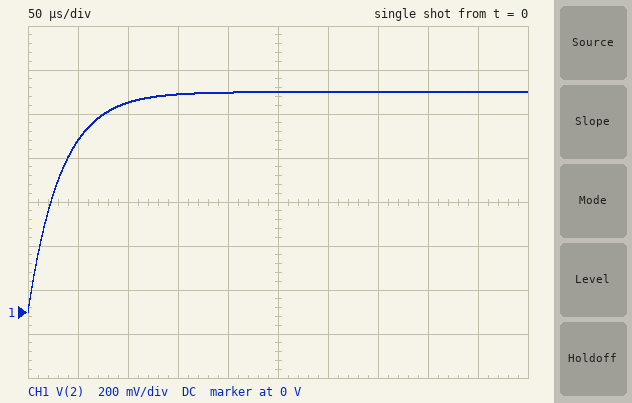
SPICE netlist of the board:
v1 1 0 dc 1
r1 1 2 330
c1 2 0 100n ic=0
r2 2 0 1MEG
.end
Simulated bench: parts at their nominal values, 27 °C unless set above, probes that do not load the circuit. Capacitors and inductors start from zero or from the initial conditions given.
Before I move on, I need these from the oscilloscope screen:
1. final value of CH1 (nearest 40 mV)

1.00 V
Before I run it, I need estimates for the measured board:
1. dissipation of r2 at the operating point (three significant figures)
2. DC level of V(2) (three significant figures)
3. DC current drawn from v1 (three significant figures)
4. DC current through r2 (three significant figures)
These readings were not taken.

999 nW
1.00 V
1.00 µA
1.00 µA
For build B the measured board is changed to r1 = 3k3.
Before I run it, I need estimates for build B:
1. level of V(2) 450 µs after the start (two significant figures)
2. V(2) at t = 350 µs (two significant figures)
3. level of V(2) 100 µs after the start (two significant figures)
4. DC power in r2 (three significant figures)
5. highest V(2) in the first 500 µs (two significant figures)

740 mV
650 mV
260 mV
993 nW
780 mV
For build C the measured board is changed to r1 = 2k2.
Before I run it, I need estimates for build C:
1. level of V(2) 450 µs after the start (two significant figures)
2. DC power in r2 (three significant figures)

870 mV
996 nW
